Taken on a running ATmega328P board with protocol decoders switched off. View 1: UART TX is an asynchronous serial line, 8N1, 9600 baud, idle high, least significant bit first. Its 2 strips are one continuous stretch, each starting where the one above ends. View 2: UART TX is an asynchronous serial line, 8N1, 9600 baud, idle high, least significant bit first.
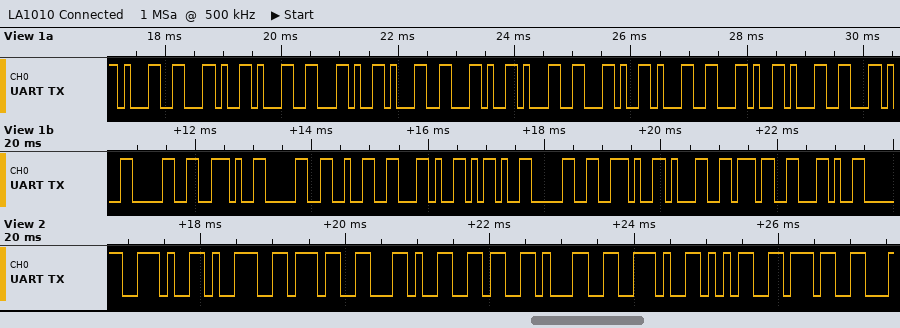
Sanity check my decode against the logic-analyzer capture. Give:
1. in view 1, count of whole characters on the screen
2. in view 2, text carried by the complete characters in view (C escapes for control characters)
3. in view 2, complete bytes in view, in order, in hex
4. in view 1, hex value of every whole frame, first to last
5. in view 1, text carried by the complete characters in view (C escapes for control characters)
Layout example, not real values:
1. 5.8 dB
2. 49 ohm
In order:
1. 23
2. ".97,61.57"
3. 2E 39 37 2C 36 31 2E 35 37
4. 31 2C 31 2C 31 2C 31 2C 31 2C 31 2C 30 2E 30 32 2C 2D 30 2E 31 37 2C
5. "1,1,1,1,1,1,0.02,-0.17,"
